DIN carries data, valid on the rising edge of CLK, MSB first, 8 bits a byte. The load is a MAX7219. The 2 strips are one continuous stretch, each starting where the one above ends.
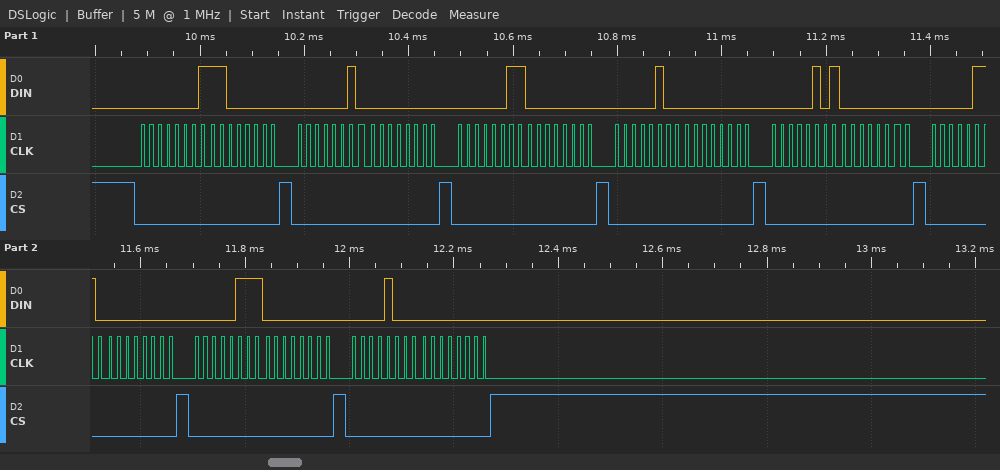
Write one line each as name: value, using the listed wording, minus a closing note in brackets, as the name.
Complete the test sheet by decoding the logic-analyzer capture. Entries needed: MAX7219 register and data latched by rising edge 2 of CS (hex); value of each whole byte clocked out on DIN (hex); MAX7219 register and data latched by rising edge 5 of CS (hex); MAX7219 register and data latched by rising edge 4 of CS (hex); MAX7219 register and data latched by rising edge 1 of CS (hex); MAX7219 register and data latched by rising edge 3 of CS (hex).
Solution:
MAX7219 register and data latched by rising edge 2 of CS: register 0x2, data 0x00
value of each whole byte clocked out on DIN: 01 C0 02 00 03 00 04 00 05 00 06 00 07 00 08 00
MAX7219 register and data latched by rising edge 5 of CS: register 0x5, data 0x00
MAX7219 register and data latched by rising edge 4 of CS: register 0x4, data 0x00
MAX7219 register and data latched by rising edge 1 of CS: register 0x1, data 0xC0
MAX7219 register and data latched by rising edge 3 of CS: register 0x3, data 0x00
